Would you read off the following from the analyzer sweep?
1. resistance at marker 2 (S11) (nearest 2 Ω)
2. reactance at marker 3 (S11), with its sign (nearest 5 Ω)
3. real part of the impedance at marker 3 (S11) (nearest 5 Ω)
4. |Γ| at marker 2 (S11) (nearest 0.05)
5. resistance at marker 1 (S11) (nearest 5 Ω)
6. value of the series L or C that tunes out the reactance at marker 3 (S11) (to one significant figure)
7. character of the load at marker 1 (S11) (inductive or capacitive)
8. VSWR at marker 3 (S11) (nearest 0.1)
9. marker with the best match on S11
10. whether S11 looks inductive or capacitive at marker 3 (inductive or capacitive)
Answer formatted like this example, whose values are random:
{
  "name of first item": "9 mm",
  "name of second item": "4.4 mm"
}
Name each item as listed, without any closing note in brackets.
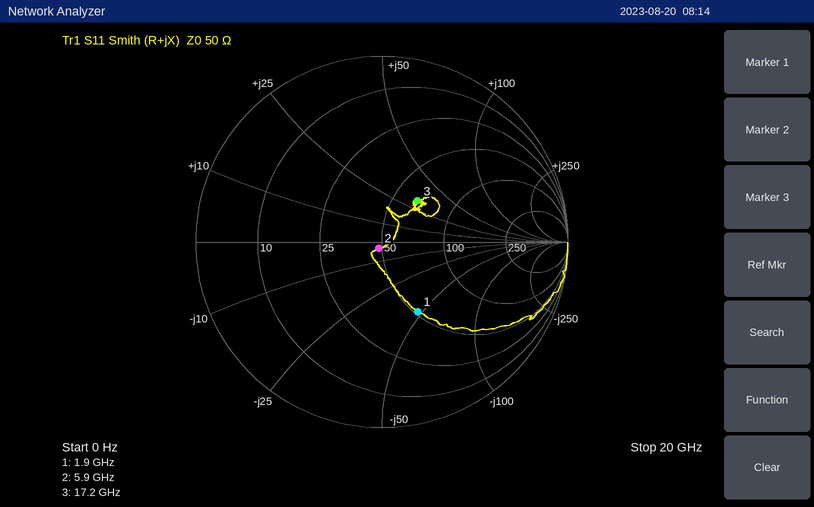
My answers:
{
  "resistance at marker 2 (S11)": "48 Ω",
  "reactance at marker 3 (S11), with its sign": "+30 Ω",
  "real part of the impedance at marker 3 (S11)": "65 Ω",
  "|Γ| at marker 2 (S11)": "0.05",
  "resistance at marker 1 (S11)": "50 Ω",
  "value of the series L or C that tunes out the reactance at marker 3 (S11)": "300 fF",
  "character of the load at marker 1 (S11)": "capacitive",
  "VSWR at marker 3 (S11)": "1.8",
  "marker with the best match on S11": "marker 2",
  "whether S11 looks inductive or capacitive at marker 3": "inductive"
}
